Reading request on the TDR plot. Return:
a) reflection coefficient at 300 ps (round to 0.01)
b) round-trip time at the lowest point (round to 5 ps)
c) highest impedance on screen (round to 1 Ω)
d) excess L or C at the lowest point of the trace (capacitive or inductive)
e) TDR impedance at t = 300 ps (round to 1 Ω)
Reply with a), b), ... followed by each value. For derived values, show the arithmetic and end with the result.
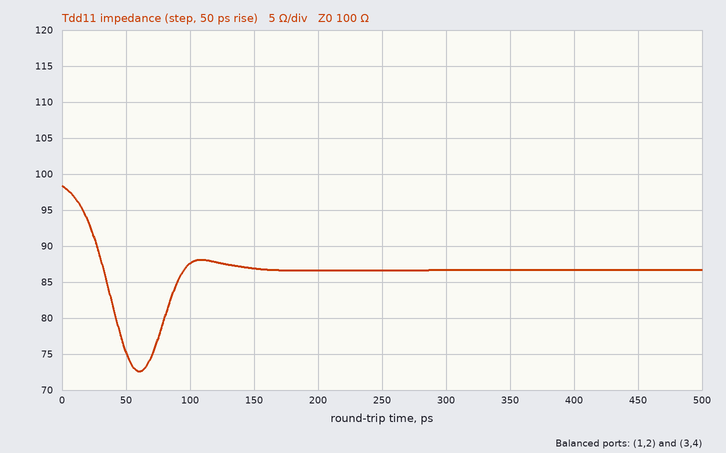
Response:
a) (87 − 100)/(87 + 100) ≈ -0.07
b) 60 ps
c) 98 Ω
d) capacitive
e) 87 Ω
